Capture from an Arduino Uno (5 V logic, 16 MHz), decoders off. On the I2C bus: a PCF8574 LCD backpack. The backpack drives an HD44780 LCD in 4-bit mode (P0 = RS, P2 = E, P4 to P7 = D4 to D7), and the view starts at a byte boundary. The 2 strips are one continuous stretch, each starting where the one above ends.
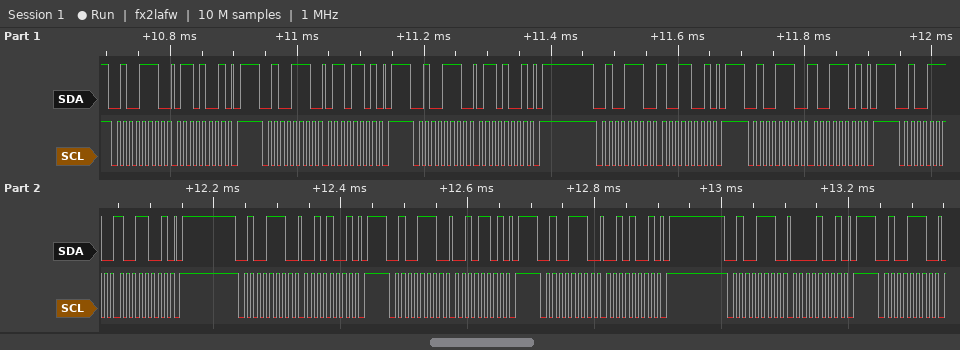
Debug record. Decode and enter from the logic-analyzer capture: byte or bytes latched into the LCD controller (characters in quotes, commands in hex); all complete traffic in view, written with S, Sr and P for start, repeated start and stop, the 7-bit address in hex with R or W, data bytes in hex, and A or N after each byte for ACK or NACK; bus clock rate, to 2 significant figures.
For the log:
'i'
S 27W A 69 A P S 27W A 6D A P S 27W A 69 A P S 27W A 99 A P S 27W A 9D A P S 27W A 99 A P S 27W A 29 A P S 27W A 2D A P S 27W A 29 A P S 27W A 09 A P S 27W A
100 kHz
